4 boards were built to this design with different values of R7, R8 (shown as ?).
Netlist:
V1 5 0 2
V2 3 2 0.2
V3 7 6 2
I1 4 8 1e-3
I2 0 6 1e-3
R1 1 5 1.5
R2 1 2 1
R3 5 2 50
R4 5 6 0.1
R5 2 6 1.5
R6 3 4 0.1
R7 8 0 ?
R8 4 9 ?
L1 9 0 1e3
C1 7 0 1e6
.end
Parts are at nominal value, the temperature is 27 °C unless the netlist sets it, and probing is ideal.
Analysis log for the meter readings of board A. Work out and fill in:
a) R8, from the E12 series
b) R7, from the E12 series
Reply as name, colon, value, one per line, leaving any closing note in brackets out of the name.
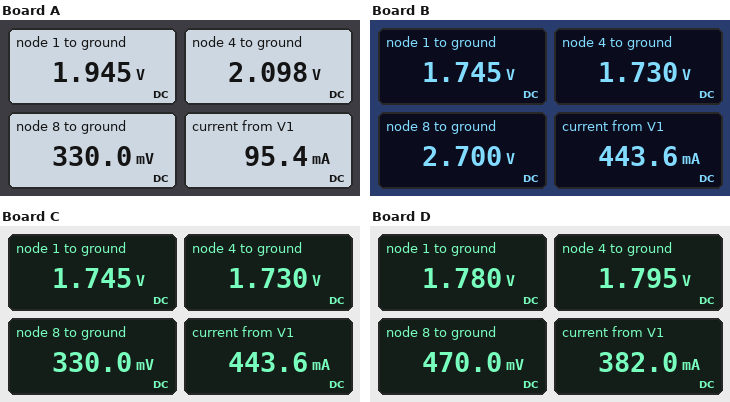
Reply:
R8, from the E12 series: 22 Ω
R7, from the E12 series: 330 Ω
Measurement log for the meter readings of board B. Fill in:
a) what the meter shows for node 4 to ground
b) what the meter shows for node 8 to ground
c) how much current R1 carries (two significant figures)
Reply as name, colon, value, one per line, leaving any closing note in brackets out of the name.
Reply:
what the meter shows for node 4 to ground: 1.730 V
what the meter shows for node 8 to ground: 2.700 V
how much current R1 carries: 170 mA
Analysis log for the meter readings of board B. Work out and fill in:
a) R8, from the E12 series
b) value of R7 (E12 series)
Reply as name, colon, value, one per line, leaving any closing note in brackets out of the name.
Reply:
R8, from the E12 series: 3.9 Ω
value of R7: 2.7 kΩ
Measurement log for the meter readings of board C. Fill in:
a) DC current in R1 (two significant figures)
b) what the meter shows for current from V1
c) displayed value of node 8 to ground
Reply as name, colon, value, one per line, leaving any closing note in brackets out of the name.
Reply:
DC current in R1: 170 mA
what the meter shows for current from V1: 443.6 mA
displayed value of node 8 to ground: 330.0 mV
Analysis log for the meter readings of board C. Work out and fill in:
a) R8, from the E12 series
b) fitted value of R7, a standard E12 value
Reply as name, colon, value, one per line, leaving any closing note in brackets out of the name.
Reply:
R8, from the E12 series: 3.9 Ω
fitted value of R7, a standard E12 value: 330 Ω
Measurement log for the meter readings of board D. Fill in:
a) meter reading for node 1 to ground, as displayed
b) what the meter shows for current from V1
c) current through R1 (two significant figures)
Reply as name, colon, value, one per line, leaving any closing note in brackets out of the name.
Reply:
meter reading for node 1 to ground, as displayed: 1.780 V
what the meter shows for current from V1: 382.0 mA
current through R1: 150 mA
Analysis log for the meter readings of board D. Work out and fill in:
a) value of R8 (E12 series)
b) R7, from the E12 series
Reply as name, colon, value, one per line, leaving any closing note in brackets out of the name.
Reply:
value of R8: 4.7 Ω
R7, from the E12 series: 470 Ω
